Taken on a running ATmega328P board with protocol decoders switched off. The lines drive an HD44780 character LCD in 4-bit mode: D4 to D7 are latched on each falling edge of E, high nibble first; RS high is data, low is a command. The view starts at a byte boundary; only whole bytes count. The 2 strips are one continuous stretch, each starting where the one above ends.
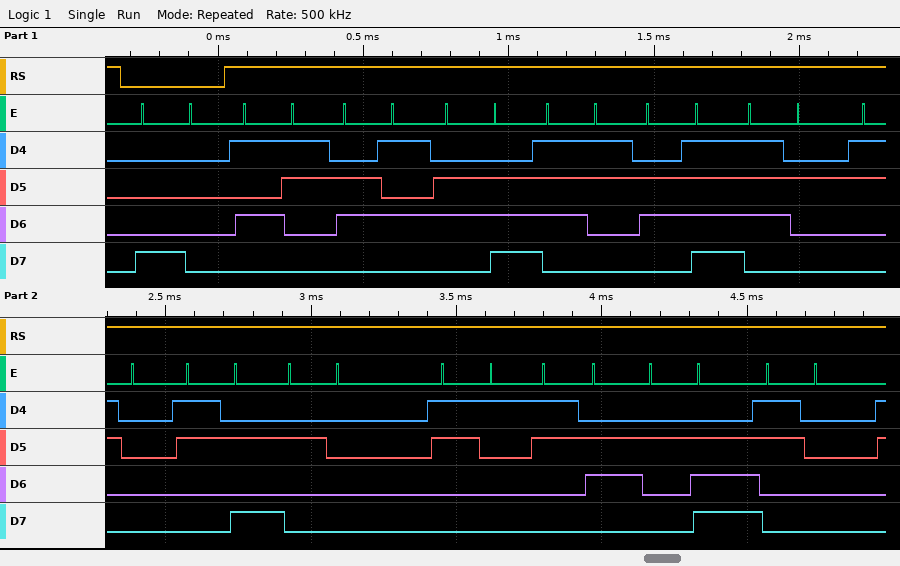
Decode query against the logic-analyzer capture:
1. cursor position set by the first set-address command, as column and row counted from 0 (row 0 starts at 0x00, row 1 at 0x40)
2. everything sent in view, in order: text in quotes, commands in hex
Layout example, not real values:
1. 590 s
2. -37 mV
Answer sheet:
1. column 0, row 0
2. 0x80 "Sensor0: 16.0"
